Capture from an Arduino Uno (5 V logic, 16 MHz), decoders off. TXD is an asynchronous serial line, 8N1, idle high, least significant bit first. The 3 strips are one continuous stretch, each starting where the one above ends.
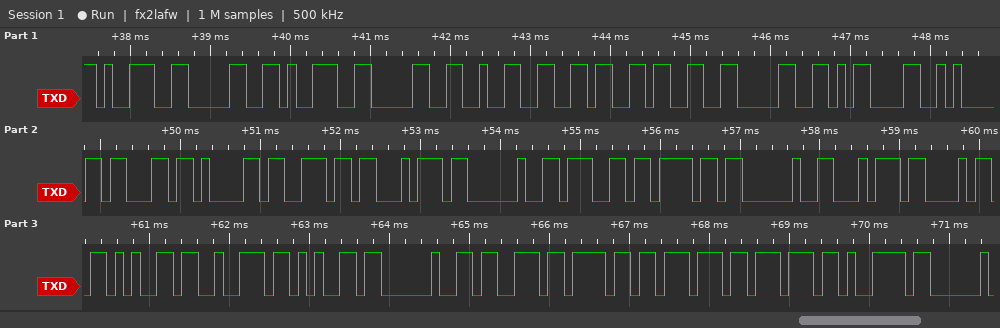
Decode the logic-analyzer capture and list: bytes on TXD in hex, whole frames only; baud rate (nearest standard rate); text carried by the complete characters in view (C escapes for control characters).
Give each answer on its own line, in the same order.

39 30 39 30 32 36 33 30 0D 0A 63 61 6E 74 20 67 6F 20 74 68 65 72 65 20 73 6F 77 77 79
9600 baud
"90902630\r\ncant go there sowwy"
